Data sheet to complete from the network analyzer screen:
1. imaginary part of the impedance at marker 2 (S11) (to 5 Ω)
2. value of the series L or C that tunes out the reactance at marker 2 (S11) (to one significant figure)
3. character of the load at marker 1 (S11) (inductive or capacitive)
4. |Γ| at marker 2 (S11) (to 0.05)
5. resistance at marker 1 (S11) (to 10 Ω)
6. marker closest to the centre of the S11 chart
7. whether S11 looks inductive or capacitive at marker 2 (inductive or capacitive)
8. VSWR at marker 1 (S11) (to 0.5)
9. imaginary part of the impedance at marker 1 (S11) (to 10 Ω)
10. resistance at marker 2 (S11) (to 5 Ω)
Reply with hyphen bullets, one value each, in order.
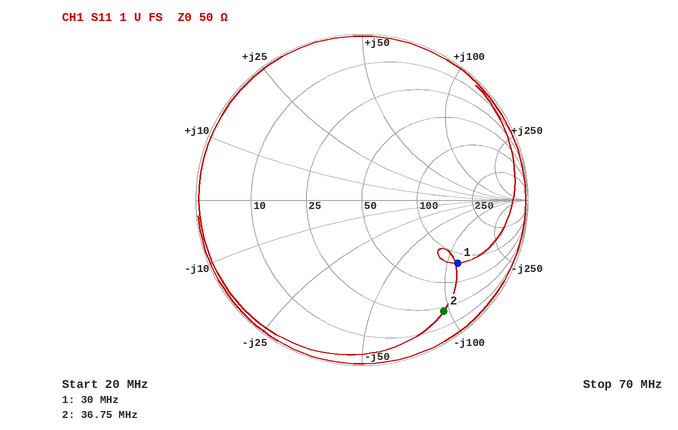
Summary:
- -95 Ω
- 400 nH
- capacitive
- 0.85
- 80 Ω
- marker 1
- capacitive
- 5.5
- -120 Ω
- 20 Ω
